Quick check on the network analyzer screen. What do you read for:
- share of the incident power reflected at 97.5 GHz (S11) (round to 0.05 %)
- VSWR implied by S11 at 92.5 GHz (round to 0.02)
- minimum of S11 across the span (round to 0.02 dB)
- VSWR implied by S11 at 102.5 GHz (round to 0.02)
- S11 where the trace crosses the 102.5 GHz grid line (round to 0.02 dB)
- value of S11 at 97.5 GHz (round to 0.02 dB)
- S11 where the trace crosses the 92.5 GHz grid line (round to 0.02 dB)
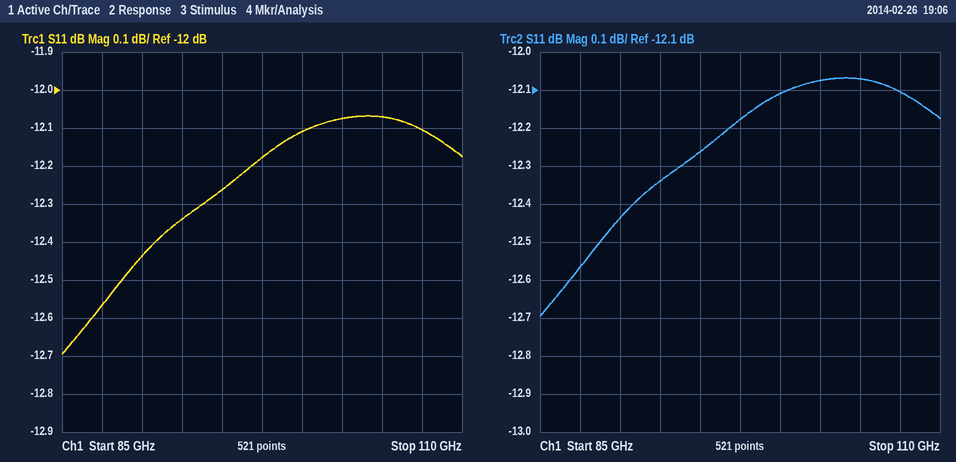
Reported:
6.05 %
1.64
-12.70 dB
1.66
-12.08 dB
-12.18 dB
-12.34 dB
